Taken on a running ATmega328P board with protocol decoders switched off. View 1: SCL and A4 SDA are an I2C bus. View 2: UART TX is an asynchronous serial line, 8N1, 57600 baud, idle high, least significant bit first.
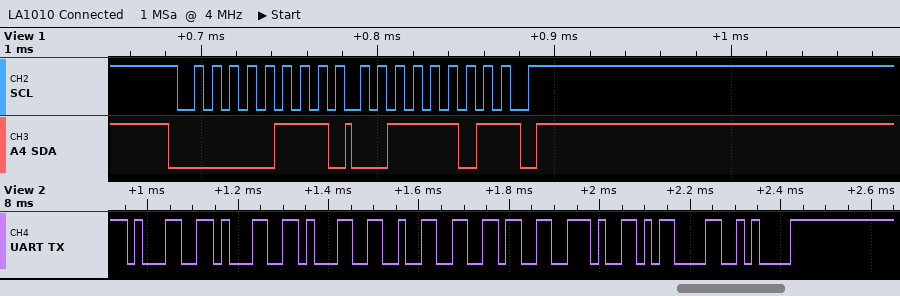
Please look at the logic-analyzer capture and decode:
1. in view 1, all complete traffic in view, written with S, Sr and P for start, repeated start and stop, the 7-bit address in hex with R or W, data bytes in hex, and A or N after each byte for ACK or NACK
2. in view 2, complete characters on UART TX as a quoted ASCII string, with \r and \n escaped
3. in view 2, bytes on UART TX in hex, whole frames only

S 03R A 3D N P
"11126.\r\n"
31 31 31 32 36 2E 0D 0A
